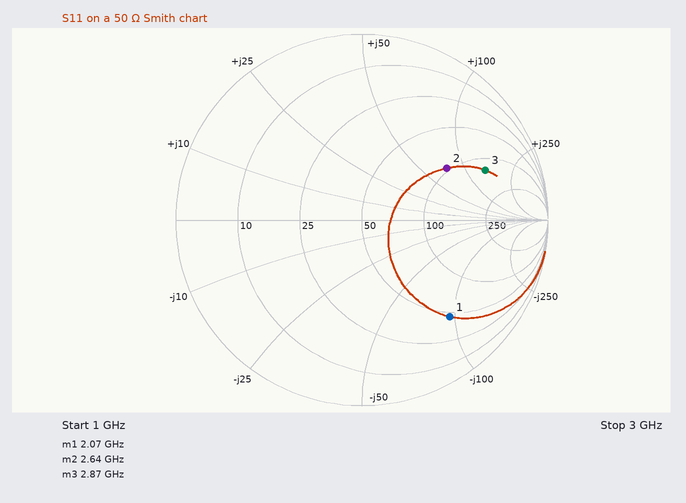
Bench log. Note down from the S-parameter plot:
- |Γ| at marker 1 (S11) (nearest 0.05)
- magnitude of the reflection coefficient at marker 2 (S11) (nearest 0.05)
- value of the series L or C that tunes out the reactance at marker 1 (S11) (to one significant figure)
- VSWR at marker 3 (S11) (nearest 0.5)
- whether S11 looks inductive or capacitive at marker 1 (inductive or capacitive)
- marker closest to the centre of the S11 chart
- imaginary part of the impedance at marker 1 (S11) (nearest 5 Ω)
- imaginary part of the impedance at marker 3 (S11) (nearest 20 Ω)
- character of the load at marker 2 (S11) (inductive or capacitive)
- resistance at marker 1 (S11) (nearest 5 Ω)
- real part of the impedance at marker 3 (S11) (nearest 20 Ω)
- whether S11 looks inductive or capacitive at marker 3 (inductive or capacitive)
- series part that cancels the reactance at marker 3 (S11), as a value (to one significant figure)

0.70
0.55
7 nH
6.0
capacitive
marker 2
-95 Ω
+140 Ω
inductive
45 Ω
140 Ω
inductive
400 fF
